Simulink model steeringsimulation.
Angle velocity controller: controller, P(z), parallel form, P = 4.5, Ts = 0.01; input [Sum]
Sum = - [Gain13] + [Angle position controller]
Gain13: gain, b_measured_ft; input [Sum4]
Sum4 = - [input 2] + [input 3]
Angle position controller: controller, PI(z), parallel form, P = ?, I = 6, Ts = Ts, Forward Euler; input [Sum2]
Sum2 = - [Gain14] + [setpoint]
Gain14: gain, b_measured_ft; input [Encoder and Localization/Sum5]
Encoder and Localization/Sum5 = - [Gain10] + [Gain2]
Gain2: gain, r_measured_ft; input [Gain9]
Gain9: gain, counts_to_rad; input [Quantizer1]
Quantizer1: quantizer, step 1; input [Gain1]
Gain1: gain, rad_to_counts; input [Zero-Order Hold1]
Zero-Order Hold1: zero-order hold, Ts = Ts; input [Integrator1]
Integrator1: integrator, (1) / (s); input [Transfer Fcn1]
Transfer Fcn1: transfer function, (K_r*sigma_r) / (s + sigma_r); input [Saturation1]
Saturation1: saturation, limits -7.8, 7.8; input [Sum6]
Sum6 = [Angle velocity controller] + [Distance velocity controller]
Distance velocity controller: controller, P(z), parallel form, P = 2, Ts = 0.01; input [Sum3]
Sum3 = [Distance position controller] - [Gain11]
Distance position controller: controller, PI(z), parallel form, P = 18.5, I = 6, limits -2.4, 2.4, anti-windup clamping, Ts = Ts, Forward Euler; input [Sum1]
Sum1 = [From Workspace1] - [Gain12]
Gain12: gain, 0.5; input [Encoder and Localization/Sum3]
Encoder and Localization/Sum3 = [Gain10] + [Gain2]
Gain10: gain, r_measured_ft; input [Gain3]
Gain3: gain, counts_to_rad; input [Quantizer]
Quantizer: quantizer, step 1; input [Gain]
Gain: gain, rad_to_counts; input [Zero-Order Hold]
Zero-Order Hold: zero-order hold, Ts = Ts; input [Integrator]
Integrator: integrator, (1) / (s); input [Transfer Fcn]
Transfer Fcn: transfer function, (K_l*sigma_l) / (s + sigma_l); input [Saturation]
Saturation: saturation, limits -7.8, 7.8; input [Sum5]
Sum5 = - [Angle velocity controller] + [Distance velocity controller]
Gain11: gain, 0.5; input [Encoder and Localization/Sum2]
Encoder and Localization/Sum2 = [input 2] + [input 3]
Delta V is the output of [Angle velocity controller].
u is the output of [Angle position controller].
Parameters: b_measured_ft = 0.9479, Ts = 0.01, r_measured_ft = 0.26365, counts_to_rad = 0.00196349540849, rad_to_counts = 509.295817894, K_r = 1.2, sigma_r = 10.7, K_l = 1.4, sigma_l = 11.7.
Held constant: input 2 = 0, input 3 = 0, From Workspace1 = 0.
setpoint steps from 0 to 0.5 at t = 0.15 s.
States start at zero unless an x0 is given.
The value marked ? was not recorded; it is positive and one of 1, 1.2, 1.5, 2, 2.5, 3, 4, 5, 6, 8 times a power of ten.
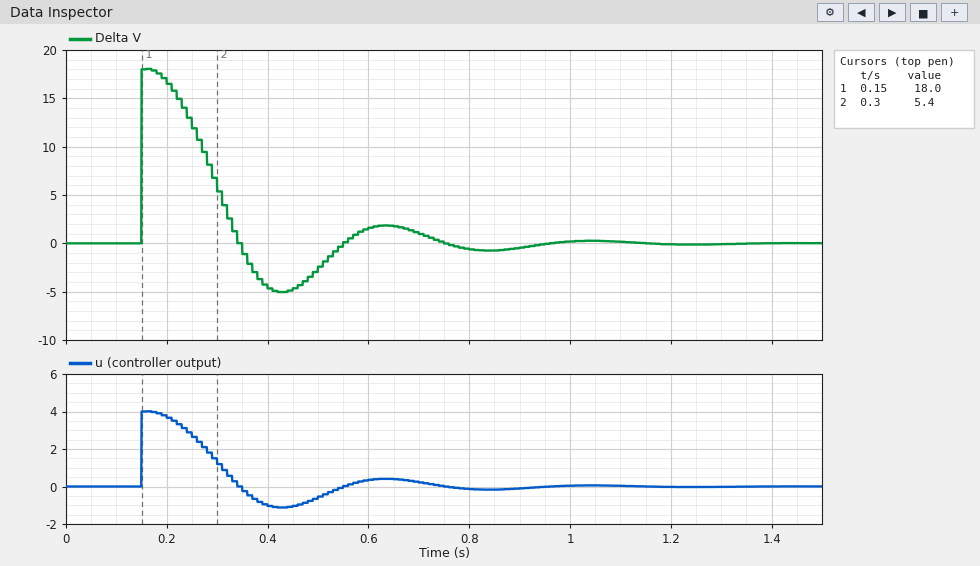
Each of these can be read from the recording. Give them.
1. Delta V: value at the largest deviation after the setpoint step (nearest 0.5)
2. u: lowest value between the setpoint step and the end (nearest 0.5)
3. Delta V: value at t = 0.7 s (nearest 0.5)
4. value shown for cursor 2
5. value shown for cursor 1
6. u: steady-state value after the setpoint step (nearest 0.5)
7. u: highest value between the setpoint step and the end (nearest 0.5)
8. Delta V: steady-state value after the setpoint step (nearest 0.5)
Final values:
18.0
-1.0
1.0
5.4
18.0
0.0
4.0
0.0
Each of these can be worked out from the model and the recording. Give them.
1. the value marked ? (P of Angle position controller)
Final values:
8
